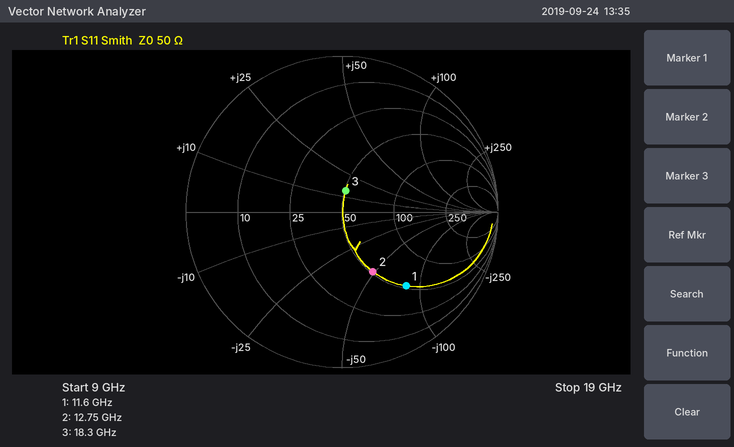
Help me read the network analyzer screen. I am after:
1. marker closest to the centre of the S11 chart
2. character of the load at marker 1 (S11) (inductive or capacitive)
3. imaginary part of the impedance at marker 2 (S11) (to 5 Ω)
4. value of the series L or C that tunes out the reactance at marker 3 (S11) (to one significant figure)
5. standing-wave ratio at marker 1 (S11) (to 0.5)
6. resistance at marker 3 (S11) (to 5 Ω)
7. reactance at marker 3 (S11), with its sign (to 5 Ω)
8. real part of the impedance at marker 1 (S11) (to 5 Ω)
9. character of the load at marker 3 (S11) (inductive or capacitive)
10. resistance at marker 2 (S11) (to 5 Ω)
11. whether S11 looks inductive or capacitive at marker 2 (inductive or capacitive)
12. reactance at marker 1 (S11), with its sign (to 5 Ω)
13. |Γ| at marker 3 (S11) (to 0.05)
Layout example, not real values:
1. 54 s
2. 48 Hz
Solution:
1. marker 3
2. capacitive
3. -50 Ω
4. 600 fF
5. 4.5
6. 50 Ω
7. +15 Ω
8. 55 Ω
9. inductive
10. 50 Ω
11. capacitive
12. -85 Ω
13. 0.15
